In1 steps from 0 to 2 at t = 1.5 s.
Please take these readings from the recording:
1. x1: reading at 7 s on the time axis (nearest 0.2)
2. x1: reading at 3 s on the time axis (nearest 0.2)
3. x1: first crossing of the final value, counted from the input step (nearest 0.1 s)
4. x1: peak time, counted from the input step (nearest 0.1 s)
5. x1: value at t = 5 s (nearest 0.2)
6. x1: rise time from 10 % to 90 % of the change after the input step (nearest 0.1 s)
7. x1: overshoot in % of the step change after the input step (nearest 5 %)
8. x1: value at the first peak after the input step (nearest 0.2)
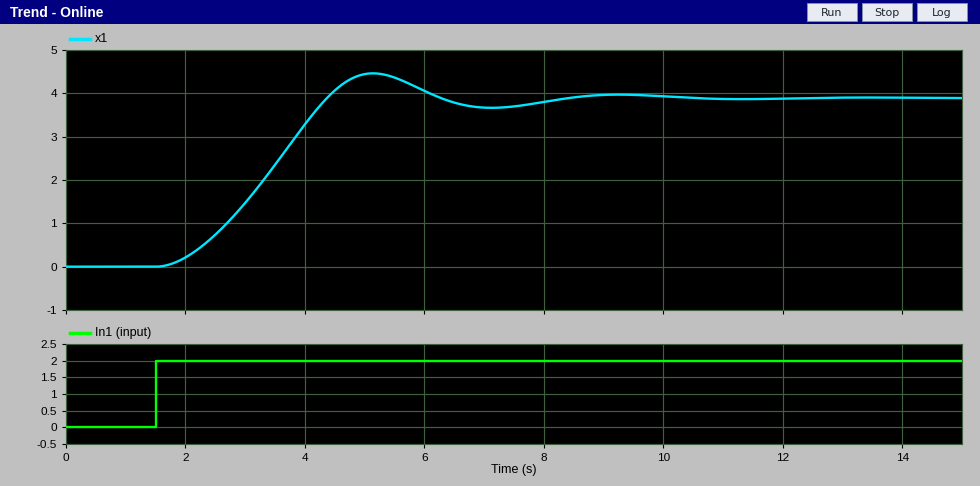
3.6
1.4
2.9 s
3.6 s
4.4
1.9 s
15 %
4.4
